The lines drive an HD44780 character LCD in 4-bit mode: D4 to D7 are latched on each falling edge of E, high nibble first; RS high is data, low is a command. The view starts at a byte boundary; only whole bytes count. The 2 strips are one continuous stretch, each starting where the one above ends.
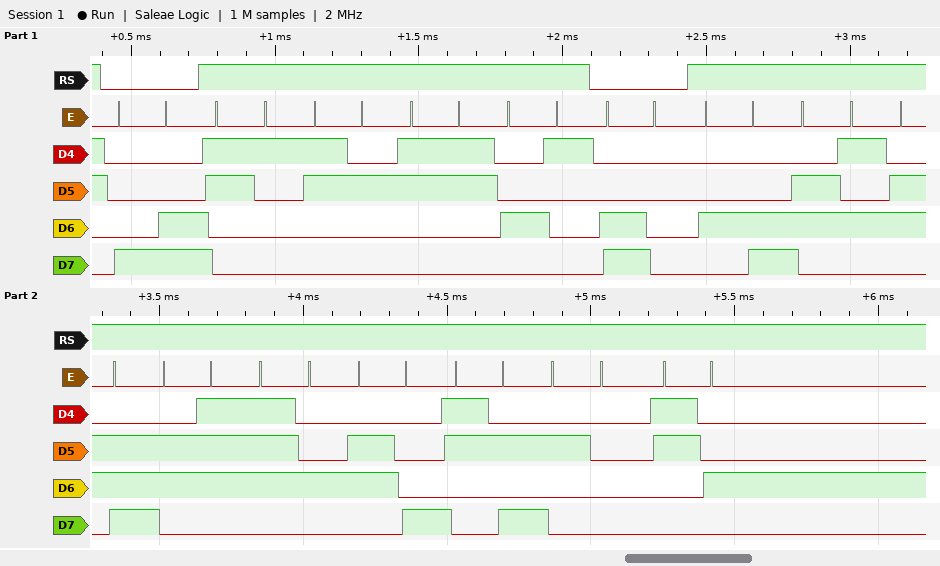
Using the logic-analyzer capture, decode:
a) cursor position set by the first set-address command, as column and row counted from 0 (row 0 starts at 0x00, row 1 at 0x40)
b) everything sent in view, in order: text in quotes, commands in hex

column 12, row 0
0x8C "123A" 0xC0 "Length: 4"
